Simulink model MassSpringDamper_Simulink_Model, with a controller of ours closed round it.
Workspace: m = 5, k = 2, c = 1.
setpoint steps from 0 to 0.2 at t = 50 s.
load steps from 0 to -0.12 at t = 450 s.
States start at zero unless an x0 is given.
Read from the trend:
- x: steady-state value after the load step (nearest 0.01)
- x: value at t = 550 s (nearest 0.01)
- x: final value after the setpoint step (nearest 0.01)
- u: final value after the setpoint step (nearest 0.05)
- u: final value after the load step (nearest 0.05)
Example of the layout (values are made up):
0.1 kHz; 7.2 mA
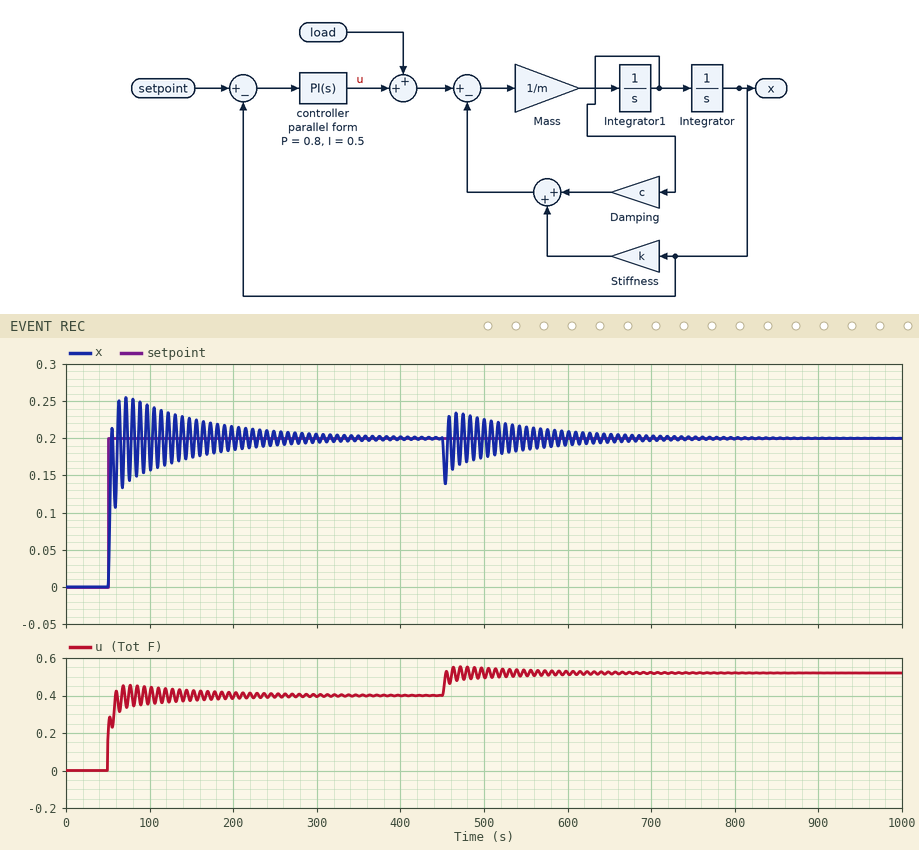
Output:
0.20; 0.21; 0.20; 0.40; 0.50
